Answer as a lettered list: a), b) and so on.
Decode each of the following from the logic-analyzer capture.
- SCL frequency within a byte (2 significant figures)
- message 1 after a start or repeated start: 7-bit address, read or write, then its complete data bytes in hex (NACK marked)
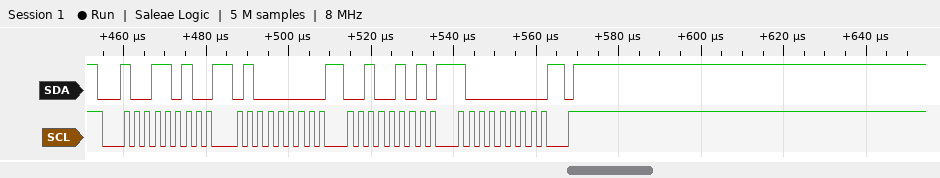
a) 400 kHz
b) 0x4D write: 40 25 80
